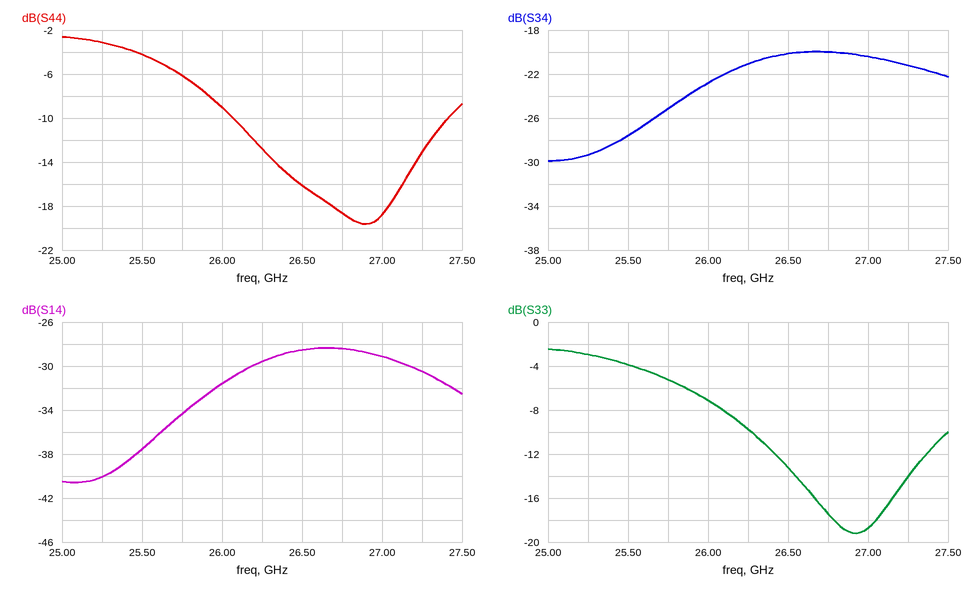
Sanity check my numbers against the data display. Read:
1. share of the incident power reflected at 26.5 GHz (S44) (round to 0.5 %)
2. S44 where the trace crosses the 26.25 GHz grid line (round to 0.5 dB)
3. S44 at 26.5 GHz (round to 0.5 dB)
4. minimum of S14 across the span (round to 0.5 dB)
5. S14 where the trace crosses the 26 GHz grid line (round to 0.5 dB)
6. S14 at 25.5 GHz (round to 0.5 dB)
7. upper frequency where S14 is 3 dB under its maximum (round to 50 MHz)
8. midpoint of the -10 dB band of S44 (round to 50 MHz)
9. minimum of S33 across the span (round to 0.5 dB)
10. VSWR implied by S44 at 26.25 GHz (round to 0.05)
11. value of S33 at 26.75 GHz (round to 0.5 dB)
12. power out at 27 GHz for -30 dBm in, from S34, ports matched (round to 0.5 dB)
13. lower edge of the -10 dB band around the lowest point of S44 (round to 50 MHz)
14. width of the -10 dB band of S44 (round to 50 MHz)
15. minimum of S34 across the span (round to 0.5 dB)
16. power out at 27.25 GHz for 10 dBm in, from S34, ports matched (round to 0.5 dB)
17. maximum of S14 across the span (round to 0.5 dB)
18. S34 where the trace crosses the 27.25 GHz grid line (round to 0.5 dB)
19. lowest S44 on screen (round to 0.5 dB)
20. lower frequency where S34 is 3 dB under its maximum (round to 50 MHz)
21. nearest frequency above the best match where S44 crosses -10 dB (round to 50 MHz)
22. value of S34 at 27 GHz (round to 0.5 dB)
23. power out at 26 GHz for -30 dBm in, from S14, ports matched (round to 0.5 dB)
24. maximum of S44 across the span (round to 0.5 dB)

2.5 %
-13.0 dB
-16.0 dB
-40.5 dB
-31.5 dB
-37.5 dB
27.35 GHz
26.75 GHz
-19.0 dB
1.60
-17.5 dB
-50.5 dBm
26.05 GHz
1.35 GHz
-30.0 dB
-11.0 dBm
-28.5 dB
-21.0 dB
-19.5 dB
26.00 GHz
27.40 GHz
-20.5 dB
-61.5 dBm
-2.5 dB
